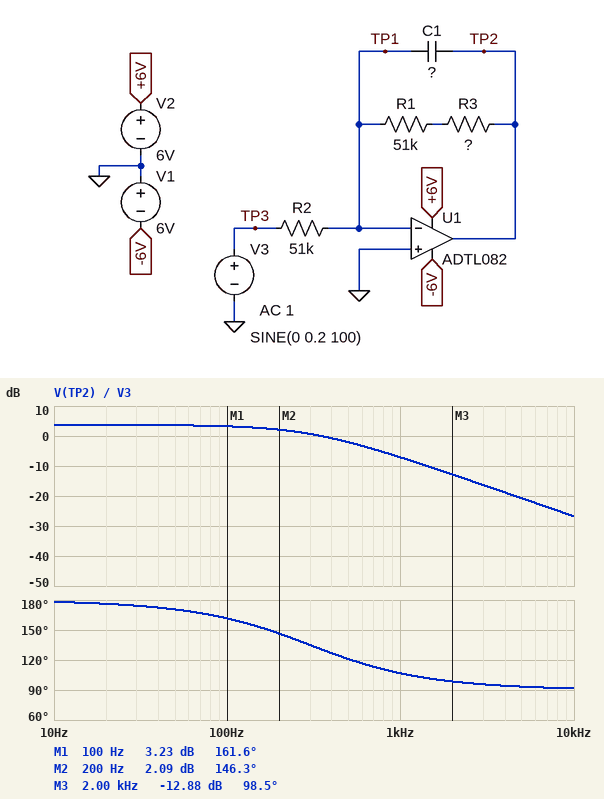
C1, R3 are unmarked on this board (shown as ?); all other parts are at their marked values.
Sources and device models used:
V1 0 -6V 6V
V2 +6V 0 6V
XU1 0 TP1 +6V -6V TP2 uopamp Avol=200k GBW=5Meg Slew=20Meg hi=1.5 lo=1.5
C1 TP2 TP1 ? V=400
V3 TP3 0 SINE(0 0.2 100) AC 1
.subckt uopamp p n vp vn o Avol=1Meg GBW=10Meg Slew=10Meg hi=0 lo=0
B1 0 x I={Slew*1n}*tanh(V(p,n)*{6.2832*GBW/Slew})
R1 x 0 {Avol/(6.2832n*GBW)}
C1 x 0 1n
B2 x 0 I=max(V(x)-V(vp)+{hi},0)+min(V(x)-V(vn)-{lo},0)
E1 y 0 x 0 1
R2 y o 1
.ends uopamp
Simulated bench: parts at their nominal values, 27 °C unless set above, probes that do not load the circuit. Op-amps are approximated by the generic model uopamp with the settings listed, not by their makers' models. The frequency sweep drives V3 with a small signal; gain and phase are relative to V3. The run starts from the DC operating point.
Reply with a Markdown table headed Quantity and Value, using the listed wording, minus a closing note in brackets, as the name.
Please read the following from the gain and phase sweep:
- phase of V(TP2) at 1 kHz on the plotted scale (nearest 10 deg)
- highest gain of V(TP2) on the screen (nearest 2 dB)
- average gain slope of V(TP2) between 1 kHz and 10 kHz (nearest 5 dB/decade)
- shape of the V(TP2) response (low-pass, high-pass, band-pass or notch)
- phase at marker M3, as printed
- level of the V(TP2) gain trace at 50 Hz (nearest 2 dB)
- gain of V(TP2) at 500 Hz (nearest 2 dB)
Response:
| Quantity | Value |
|---|---|
| phase of V(TP2) at 1 kHz on the plotted scale | 110 deg |
| highest gain of V(TP2) on the screen | 4 dB |
| average gain slope of V(TP2) between 1 kHz and 10 kHz | -20 dB/decade |
| shape of the V(TP2) response | low-pass |
| phase at marker M3, as printed | 98.5 deg |
| level of the V(TP2) gain trace at 50 Hz | 4 dB |
| gain of V(TP2) at 500 Hz | -2 dB |
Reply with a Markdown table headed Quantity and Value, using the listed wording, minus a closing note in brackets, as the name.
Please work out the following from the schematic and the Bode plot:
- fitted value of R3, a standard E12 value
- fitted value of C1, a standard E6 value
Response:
| Quantity | Value |
|---|---|
| fitted value of R3, a standard E12 value | 27 kΩ |
| fitted value of C1, a standard E6 value | 6.8 nF |
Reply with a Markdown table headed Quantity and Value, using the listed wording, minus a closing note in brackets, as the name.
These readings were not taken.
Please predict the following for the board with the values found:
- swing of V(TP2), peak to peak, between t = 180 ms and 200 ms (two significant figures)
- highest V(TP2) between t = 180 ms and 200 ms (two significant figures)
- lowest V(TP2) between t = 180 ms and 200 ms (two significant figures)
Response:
| Quantity | Value |
|---|---|
| swing of V(TP2), peak to peak, between t = 180 ms and 200 ms | 580 mV |
| highest V(TP2) between t = 180 ms and 200 ms | 290 mV |
| lowest V(TP2) between t = 180 ms and 200 ms | -290 mV |
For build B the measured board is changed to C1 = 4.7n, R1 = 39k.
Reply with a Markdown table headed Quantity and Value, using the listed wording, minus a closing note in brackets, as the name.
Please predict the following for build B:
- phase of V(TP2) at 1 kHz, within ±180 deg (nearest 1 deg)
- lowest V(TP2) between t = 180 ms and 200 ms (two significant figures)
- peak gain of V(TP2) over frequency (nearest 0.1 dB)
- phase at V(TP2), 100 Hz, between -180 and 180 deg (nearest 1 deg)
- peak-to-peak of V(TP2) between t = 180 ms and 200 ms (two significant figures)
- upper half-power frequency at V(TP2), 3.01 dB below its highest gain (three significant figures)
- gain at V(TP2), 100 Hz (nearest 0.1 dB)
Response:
| Quantity | Value |
|---|---|
| phase of V(TP2) at 1 kHz, within ±180 deg | 117 deg |
| lowest V(TP2) between t = 180 ms and 200 ms | -250 mV |
| peak gain of V(TP2) over frequency | 2.2 dB |
| phase at V(TP2), 100 Hz, between -180 and 180 deg | 169 deg |
| peak-to-peak of V(TP2) between t = 180 ms and 200 ms | 510 mV |
| upper half-power frequency at V(TP2), 3.01 dB below its highest gain | 513 Hz |
| gain at V(TP2), 100 Hz | 2.1 dB |
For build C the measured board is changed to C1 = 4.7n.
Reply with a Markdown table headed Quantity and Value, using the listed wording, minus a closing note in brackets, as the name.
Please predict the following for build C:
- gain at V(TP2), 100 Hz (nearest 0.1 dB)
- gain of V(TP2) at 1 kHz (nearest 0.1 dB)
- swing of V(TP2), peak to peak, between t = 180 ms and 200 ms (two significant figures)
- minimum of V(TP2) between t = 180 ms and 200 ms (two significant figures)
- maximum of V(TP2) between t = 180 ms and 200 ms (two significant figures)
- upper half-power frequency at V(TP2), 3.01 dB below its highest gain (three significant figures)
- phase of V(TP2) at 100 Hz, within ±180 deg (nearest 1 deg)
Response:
| Quantity | Value |
|---|---|
| gain at V(TP2), 100 Hz | 3.5 dB |
| gain of V(TP2) at 1 kHz | -4.3 dB |
| swing of V(TP2), peak to peak, between t = 180 ms and 200 ms | 600 mV |
| minimum of V(TP2) between t = 180 ms and 200 ms | -300 mV |
| maximum of V(TP2) between t = 180 ms and 200 ms | 300 mV |
| upper half-power frequency at V(TP2), 3.01 dB below its highest gain | 434 Hz |
| phase of V(TP2) at 100 Hz, within ±180 deg | 167 deg |
